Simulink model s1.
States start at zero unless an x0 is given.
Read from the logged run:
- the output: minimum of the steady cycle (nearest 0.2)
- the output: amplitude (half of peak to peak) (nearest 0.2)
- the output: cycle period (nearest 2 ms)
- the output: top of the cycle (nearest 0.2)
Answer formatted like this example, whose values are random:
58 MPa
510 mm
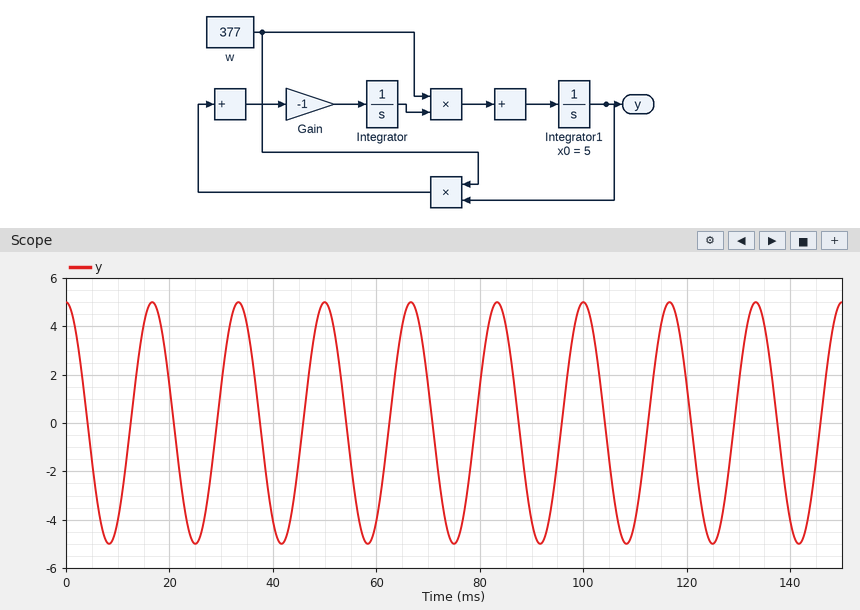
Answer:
-5.0
5.0
16 ms
5.0
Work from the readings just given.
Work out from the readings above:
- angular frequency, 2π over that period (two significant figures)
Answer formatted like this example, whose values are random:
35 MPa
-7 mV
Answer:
0.39 rad/ms
